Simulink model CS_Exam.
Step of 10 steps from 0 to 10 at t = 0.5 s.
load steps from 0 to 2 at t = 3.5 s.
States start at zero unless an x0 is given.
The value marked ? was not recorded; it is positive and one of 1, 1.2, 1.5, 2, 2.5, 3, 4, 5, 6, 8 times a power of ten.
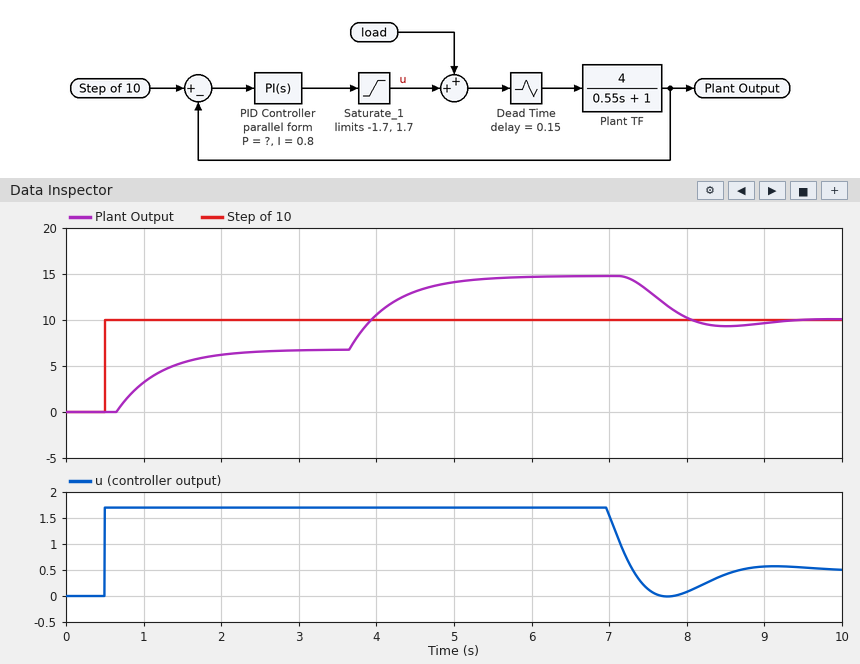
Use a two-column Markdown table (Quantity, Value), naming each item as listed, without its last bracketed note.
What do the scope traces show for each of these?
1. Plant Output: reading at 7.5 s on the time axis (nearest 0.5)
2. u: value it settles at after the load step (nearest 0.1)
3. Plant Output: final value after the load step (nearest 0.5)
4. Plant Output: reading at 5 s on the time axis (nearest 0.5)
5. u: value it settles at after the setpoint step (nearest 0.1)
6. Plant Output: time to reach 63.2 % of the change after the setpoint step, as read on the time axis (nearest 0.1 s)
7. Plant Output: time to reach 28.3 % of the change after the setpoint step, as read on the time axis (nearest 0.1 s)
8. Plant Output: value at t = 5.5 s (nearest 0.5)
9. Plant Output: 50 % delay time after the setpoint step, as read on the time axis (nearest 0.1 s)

| Quantity | Value |
|---|---|
| Plant Output: reading at 7.5 s on the time axis | 13.0 |
| u: value it settles at after the load step | 0.5 |
| Plant Output: final value after the load step | 10.0 |
| Plant Output: reading at 5 s on the time axis | 14.0 |
| u: value it settles at after the setpoint step | 1.7 |
| Plant Output: time to reach 63.2 % of the change after the setpoint step, as read on the time axis | 1.2 s |
| Plant Output: time to reach 28.3 % of the change after the setpoint step, as read on the time axis | 0.8 s |
| Plant Output: value at t = 5.5 s | 14.5 |
| Plant Output: 50 % delay time after the setpoint step, as read on the time axis | 1.0 s |
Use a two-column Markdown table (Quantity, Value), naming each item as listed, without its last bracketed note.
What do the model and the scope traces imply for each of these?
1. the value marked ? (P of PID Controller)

| Quantity | Value |
|---|---|
| the value marked ? | 0.2 |
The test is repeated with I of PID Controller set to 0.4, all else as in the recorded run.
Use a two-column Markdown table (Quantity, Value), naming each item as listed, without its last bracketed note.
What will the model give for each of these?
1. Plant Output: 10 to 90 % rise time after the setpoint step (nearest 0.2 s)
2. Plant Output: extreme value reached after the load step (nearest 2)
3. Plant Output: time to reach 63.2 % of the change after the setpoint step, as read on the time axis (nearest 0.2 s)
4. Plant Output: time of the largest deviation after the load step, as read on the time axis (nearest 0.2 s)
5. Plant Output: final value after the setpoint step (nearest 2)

| Quantity | Value |
|---|---|
| Plant Output: 10 to 90 % rise time after the setpoint step | 1.2 s |
| Plant Output: extreme value reached after the load step | 14 |
| Plant Output: time to reach 63.2 % of the change after the setpoint step, as read on the time axis | 1.2 s |
| Plant Output: time of the largest deviation after the load step, as read on the time axis | 6.4 s |
| Plant Output: final value after the setpoint step | 6 |
